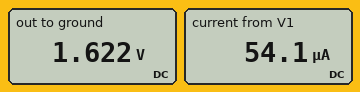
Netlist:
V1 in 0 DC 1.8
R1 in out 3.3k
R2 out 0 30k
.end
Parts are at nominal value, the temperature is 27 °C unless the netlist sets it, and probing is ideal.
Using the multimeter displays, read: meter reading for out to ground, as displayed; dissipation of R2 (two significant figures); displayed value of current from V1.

1.622 V
88 µW
54.1 µA
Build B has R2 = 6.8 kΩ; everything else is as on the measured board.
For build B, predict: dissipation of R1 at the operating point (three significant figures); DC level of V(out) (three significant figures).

105 µW
1.21 V
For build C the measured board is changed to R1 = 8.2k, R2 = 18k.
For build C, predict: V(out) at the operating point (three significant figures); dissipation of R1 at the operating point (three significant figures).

1.24 V
38.7 µW
